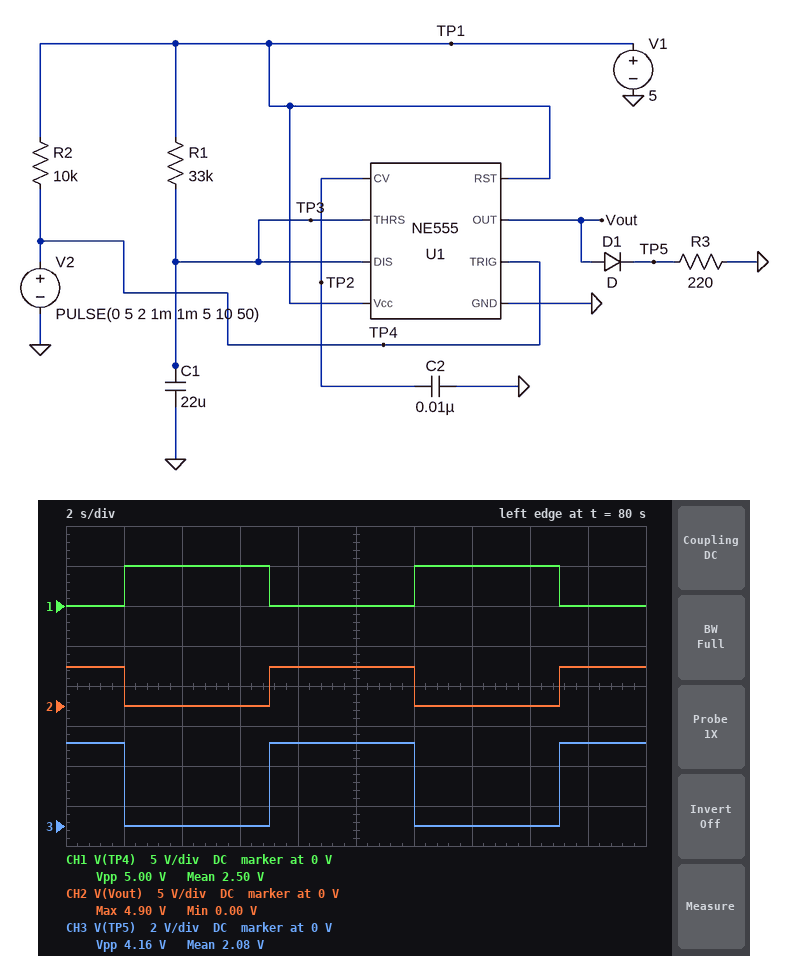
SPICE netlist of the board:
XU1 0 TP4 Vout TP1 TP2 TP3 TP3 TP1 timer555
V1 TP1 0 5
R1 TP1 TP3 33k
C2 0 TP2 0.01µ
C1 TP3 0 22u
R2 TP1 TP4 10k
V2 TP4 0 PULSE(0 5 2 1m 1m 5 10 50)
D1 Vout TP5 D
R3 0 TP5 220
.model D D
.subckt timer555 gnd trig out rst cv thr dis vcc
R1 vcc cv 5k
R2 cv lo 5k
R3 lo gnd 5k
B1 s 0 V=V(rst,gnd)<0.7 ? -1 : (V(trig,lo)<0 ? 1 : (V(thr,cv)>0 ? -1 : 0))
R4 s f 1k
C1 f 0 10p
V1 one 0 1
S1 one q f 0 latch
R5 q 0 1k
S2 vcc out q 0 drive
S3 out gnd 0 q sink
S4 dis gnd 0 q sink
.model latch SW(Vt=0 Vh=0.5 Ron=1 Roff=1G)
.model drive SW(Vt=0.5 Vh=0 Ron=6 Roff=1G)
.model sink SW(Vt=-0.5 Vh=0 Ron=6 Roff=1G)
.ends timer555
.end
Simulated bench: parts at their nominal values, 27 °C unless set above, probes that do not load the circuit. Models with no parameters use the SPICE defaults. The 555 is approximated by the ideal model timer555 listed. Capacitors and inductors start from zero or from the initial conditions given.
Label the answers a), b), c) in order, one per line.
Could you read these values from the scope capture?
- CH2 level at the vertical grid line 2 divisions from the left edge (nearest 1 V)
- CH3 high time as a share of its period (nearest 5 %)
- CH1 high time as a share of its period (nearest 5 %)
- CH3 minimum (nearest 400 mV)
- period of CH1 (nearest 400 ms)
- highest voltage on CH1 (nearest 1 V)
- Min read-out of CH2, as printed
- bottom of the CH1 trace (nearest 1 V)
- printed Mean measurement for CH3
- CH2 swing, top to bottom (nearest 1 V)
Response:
a) 0 V
b) 50 %
c) 50 %
d) 0 V
e) 10.0 s
f) 5 V
g) 0.00 V
h) 0 V
i) 2.08 V
j) 5 V
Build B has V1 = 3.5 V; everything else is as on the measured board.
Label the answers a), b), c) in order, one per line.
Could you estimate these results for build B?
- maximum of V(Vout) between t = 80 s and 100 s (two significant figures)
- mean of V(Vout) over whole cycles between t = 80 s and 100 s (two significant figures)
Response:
a) 3.4 V
b) 1.7 V
